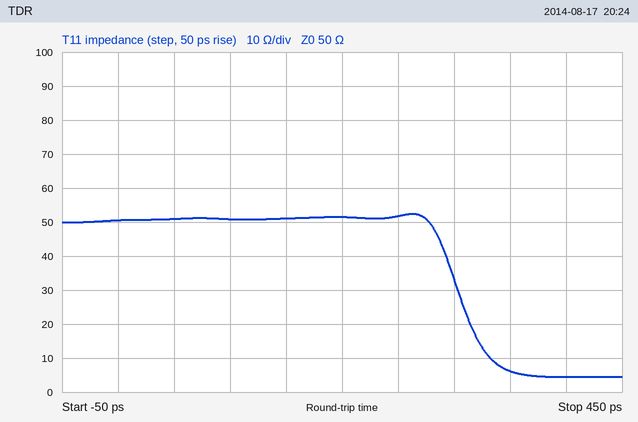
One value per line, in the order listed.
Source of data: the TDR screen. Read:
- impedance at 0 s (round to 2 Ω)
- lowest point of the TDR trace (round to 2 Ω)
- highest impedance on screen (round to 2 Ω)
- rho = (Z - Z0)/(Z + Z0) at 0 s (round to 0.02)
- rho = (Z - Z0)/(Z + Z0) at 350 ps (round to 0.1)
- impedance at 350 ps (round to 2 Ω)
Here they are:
50 Ω
4 Ω
52 Ω
0.00
-0.8
6 Ω
